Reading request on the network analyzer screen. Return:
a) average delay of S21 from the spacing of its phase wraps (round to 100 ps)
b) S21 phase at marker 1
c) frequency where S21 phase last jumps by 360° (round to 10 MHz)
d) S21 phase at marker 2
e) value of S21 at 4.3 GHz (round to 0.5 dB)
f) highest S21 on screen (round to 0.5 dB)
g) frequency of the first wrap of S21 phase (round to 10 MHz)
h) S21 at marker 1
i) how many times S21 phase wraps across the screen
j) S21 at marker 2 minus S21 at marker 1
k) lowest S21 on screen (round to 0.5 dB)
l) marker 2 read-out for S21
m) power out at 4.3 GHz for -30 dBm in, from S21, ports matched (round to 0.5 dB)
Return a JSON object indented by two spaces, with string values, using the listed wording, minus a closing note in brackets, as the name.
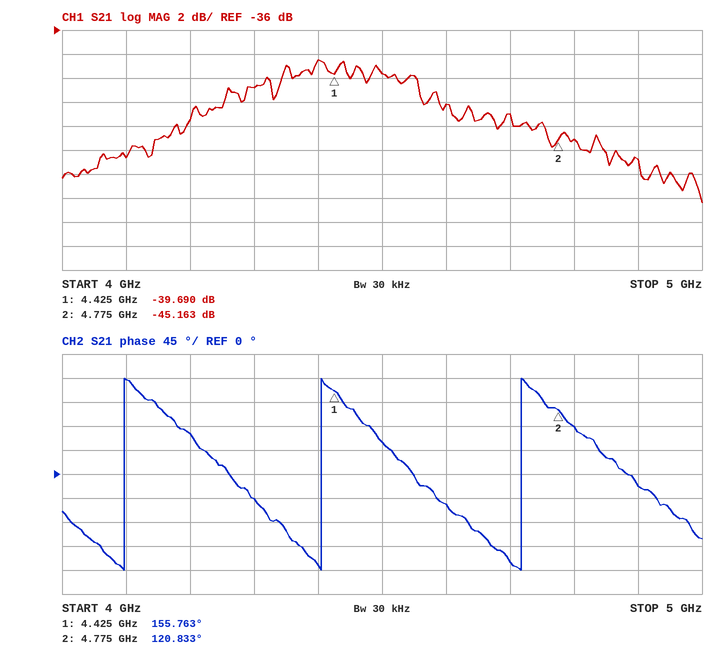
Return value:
{
  "average delay of S21 from the spacing of its phase wraps": "3.2 ns",
  "S21 phase at marker 1": "155.763°",
  "frequency where S21 phase last jumps by 360°": "4.72 GHz",
  "S21 phase at marker 2": "120.833°",
  "value of S21 at 4.3 GHz": "-41.0 dB",
  "highest S21 on screen": "-38.5 dB",
  "frequency of the first wrap of S21 phase": "4.10 GHz",
  "S21 at marker 1": "-39.690 dB",
  "how many times S21 phase wraps across the screen": "3",
  "S21 at marker 2 minus S21 at marker 1": "-5.473 dB",
  "lowest S21 on screen": "-50.5 dB",
  "marker 2 read-out for S21": "-45.163 dB",
  "power out at 4.3 GHz for -30 dBm in, from S21, ports matched": "-71.0 dBm"
}
